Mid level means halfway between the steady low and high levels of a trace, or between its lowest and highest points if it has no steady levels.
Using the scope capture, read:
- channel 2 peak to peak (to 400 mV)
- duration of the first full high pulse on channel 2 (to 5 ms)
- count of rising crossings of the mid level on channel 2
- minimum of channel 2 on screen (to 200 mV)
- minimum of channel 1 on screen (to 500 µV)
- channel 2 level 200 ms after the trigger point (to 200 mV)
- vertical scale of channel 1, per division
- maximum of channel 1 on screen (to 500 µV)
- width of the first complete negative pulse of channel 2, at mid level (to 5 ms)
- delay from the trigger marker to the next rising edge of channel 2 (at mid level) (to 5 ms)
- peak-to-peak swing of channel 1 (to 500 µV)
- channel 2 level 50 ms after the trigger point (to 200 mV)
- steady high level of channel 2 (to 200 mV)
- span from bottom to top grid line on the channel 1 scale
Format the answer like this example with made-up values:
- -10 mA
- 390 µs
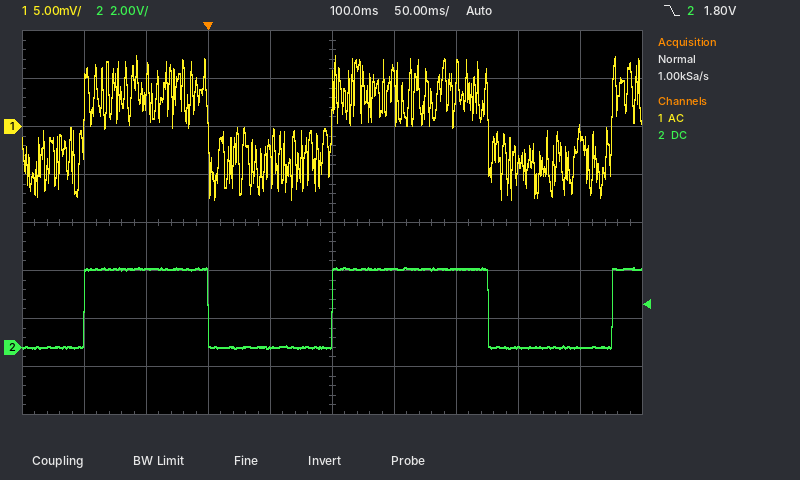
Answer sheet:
- 3.2 V
- 100 ms
- 3
- 0.0 V
- -7.5 mV
- 3.2 V
- 5 mV
- 7.5 mV
- 100 ms
- 100 ms
- 15.0 mV
- 0.0 V
- 3.2 V
- 40 mV
